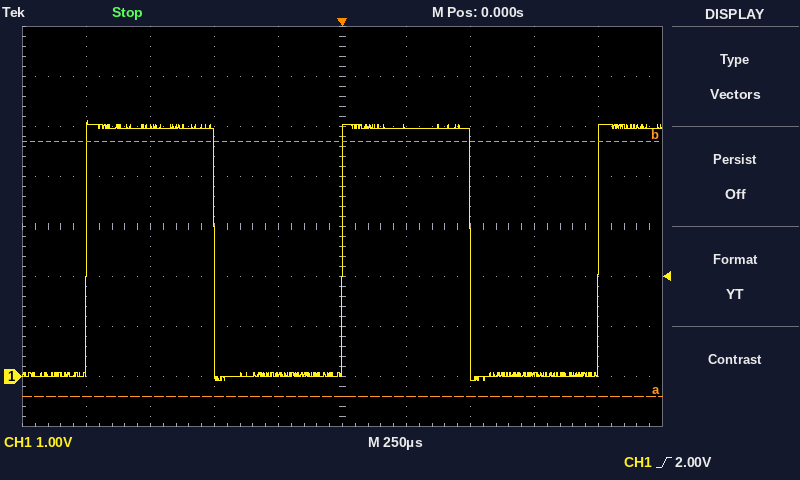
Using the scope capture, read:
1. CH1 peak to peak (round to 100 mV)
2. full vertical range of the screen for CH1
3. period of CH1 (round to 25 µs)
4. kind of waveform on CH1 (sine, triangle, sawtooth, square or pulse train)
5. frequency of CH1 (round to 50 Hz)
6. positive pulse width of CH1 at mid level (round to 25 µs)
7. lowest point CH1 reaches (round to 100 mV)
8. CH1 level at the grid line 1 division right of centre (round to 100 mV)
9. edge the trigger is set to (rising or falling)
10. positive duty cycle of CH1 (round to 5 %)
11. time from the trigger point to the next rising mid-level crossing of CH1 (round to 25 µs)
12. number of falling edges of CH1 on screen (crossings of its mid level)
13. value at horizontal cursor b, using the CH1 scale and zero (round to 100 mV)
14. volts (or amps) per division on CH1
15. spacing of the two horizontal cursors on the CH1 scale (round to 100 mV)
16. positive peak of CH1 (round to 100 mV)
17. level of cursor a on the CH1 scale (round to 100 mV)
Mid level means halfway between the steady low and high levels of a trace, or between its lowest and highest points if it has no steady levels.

5.2 V
8 V
1.000 ms
square
1.00 kHz
500 µs
-100 mV
5.0 V
rising
50 %
1.000 ms
2
4.7 V
1 V
5.1 V
5.1 V
-400 mV
